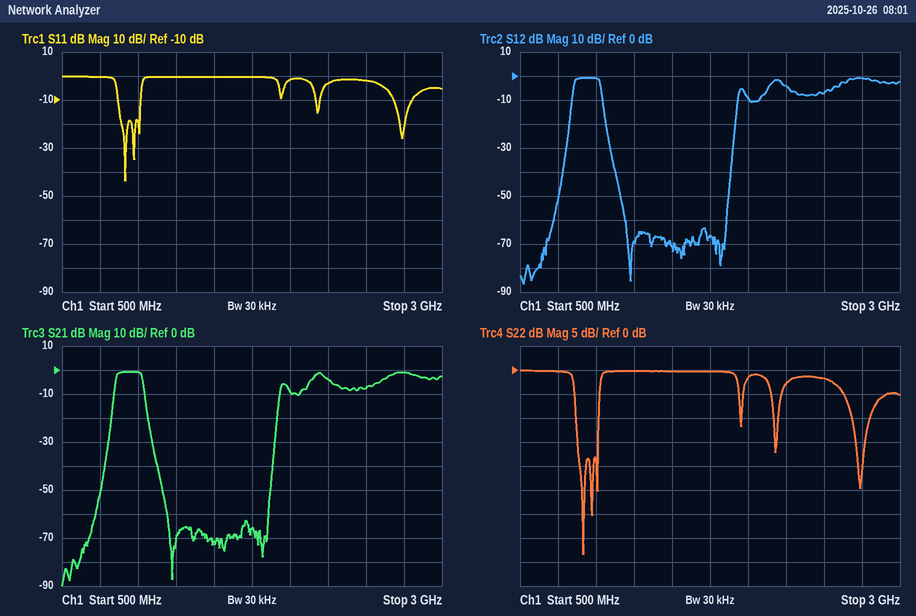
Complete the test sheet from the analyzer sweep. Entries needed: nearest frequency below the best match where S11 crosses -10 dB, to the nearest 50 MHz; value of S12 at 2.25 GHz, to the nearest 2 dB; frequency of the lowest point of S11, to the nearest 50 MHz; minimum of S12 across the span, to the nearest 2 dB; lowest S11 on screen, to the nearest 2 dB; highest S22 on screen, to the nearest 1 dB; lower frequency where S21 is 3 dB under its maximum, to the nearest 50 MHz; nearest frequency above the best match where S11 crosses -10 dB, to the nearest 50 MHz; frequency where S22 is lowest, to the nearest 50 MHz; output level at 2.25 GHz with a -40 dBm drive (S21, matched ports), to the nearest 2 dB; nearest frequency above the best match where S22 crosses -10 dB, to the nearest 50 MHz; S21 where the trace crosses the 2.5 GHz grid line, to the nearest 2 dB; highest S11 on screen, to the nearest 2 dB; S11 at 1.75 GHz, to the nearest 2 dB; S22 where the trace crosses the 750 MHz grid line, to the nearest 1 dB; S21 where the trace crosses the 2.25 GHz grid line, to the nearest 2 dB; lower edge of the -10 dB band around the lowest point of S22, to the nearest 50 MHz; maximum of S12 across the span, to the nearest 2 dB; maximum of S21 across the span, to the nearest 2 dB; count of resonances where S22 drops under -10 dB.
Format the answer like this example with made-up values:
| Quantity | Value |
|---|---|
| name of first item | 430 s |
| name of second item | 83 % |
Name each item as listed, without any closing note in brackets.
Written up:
| Quantity | Value |
|---|---|
| nearest frequency below the best match where S11 crosses -10 dB, to the nearest 50 MHz | 850 MHz |
| value of S12 at 2.25 GHz, to the nearest 2 dB | -4 dB |
| frequency of the lowest point of S11, to the nearest 50 MHz | 900 MHz |
| minimum of S12 across the span, to the nearest 2 dB | -86 dB |
| lowest S11 on screen, to the nearest 2 dB | -44 dB |
| highest S22 on screen, to the nearest 1 dB | 0 dB |
| lower frequency where S21 is 3 dB under its maximum, to the nearest 50 MHz | 850 MHz |
| nearest frequency above the best match where S11 crosses -10 dB, to the nearest 50 MHz | 1.00 GHz |
| frequency where S22 is lowest, to the nearest 50 MHz | 900 MHz |
| output level at 2.25 GHz with a -40 dBm drive (S21, matched ports), to the nearest 2 dB | -44 dBm |
| nearest frequency above the best match where S22 crosses -10 dB, to the nearest 50 MHz | 1.00 GHz |
| S21 where the trace crosses the 2.5 GHz grid line, to the nearest 2 dB | -8 dB |
| highest S11 on screen, to the nearest 2 dB | 0 dB |
| S11 at 1.75 GHz, to the nearest 2 dB | 0 dB |
| S22 where the trace crosses the 750 MHz grid line, to the nearest 1 dB | 0 dB |
| S21 where the trace crosses the 2.25 GHz grid line, to the nearest 2 dB | -4 dB |
| lower edge of the -10 dB band around the lowest point of S22, to the nearest 50 MHz | 850 MHz |
| maximum of S12 across the span, to the nearest 2 dB | 0 dB |
| maximum of S21 across the span, to the nearest 2 dB | 0 dB |
| count of resonances where S22 drops under -10 dB | 6 |
